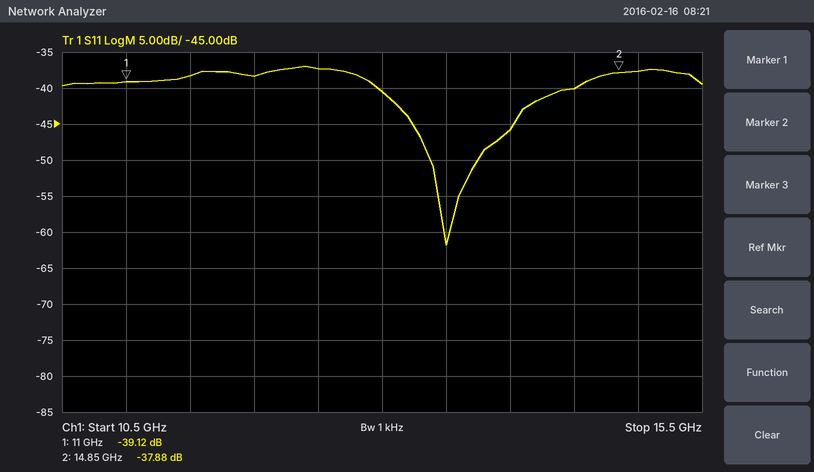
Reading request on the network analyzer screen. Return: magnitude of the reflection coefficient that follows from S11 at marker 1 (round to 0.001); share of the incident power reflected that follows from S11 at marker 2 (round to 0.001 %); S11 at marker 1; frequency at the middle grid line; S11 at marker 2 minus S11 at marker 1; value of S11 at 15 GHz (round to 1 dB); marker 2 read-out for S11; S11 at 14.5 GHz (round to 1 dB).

0.011
0.016 %
-39.12 dB
13 GHz
1.24 dB
-38 dB
-37.88 dB
-40 dB
